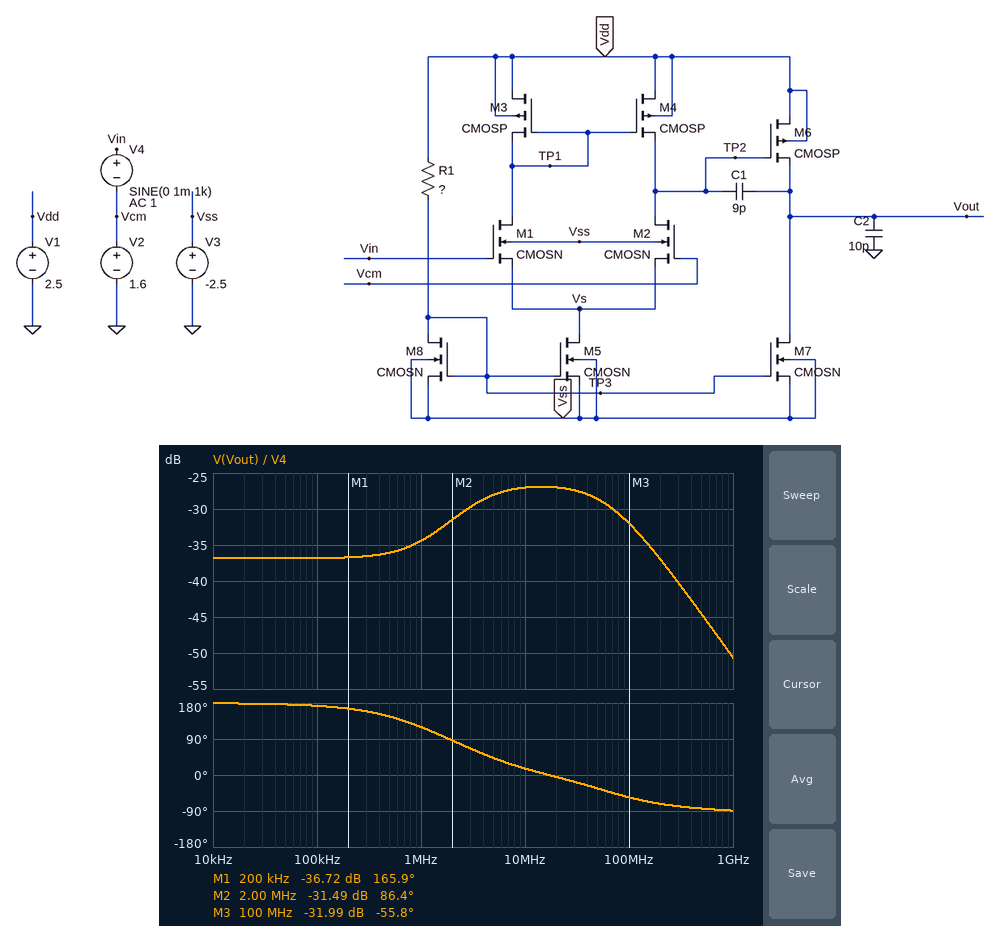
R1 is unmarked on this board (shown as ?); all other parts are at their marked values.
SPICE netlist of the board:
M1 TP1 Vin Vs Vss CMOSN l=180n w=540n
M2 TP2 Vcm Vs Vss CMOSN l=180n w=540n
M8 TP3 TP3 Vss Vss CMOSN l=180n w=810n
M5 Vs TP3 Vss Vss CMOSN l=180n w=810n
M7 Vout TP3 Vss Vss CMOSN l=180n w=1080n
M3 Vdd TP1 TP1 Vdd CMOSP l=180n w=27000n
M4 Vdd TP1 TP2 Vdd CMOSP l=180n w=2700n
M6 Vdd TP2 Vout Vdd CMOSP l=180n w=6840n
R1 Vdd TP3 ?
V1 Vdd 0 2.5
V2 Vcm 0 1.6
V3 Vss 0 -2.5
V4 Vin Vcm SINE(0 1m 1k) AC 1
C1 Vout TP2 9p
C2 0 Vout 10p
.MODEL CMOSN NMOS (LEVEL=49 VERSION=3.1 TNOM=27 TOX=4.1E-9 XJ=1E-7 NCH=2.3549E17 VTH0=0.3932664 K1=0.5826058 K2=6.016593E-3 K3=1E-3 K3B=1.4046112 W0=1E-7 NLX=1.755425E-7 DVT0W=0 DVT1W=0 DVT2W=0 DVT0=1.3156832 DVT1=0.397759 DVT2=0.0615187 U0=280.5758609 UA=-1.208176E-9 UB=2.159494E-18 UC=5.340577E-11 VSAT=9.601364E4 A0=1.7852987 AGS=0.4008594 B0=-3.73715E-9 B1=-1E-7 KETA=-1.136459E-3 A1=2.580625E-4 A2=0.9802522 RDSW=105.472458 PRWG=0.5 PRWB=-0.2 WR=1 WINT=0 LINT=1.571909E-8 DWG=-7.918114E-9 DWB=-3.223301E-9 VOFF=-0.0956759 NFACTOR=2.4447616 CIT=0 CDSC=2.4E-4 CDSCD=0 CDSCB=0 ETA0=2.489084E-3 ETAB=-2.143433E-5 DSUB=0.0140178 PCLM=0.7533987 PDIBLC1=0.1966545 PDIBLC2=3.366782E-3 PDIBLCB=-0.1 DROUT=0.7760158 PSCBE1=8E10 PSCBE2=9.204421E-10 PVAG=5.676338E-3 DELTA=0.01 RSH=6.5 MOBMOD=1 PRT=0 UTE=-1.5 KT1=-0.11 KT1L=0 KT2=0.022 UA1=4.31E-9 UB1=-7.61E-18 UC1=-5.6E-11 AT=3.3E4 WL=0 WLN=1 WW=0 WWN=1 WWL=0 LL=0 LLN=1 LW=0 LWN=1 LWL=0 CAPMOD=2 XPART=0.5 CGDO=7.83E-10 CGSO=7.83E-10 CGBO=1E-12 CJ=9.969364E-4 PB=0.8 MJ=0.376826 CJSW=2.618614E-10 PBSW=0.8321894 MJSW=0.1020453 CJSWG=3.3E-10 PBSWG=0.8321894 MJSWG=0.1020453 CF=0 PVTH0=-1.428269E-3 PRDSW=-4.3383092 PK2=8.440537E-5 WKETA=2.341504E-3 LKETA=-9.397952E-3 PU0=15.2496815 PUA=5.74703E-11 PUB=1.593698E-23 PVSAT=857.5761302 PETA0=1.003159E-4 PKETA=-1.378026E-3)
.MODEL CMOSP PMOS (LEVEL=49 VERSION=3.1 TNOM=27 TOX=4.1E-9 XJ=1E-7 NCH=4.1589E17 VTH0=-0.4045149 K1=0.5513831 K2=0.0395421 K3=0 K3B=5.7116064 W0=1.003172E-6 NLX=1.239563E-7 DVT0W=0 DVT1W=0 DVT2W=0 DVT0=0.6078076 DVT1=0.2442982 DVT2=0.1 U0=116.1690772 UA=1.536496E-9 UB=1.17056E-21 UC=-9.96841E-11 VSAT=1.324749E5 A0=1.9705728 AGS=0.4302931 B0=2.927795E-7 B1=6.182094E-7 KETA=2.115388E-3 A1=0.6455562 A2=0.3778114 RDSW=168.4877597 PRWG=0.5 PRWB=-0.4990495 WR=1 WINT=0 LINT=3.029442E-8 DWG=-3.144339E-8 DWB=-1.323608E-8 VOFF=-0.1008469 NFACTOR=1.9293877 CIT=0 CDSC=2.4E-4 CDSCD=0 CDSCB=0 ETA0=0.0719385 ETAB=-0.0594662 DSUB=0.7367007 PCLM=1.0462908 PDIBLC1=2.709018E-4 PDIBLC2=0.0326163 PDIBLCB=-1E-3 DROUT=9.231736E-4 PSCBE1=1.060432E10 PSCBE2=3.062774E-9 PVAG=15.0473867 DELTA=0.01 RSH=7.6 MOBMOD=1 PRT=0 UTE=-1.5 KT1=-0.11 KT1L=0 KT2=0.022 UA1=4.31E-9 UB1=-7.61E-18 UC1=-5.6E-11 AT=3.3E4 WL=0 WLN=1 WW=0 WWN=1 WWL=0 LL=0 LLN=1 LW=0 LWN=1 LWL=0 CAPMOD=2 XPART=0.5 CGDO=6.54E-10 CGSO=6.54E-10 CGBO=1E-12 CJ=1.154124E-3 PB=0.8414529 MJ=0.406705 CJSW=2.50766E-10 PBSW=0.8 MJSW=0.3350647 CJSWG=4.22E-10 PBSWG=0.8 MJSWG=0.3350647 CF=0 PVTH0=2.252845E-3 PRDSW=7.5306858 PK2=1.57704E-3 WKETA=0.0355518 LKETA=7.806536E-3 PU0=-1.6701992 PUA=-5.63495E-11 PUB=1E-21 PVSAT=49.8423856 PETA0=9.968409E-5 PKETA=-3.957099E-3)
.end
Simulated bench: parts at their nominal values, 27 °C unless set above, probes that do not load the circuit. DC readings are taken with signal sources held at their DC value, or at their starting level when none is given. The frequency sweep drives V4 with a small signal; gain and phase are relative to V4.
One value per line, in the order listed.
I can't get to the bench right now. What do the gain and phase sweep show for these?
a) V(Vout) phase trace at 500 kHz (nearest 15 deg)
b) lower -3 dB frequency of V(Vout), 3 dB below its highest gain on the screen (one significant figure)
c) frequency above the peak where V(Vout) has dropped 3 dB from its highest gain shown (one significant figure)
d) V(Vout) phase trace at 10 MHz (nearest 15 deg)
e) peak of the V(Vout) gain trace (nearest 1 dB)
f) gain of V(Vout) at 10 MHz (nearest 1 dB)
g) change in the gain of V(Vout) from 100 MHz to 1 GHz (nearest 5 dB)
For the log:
150 deg
3 MHz
70 MHz
15 deg
-27 dB
-27 dB
-20 dB
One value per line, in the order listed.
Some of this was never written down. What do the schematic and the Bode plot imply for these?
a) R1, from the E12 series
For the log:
33 kΩ
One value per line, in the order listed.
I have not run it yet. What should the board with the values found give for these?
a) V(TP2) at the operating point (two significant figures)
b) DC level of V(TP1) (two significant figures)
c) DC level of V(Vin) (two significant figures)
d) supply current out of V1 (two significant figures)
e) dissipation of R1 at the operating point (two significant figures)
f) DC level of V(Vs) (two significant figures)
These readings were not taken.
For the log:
140 mV
1.9 V
1.6 V
510 µA
500 µW
80 mV
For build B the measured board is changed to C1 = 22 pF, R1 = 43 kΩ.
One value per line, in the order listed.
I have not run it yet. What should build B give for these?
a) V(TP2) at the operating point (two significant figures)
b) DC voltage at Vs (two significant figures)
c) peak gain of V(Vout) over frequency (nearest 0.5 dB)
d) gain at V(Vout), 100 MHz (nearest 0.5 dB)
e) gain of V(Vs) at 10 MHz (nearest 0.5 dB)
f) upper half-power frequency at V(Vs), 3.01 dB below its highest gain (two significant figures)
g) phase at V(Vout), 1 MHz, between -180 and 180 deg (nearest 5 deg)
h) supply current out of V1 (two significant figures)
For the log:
200 mV
150 mV
-27.0 dB
-32.5 dB
-7.5 dB
1.9 MHz
75 deg
420 µA
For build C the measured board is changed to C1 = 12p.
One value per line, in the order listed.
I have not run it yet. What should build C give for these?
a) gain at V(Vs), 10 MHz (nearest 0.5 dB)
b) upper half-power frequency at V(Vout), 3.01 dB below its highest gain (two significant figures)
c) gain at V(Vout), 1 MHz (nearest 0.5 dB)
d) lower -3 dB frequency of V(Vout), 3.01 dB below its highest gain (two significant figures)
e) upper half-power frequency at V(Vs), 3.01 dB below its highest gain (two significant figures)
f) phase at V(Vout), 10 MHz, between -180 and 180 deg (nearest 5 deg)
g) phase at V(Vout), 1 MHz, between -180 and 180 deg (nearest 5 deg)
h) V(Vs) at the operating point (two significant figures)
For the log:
-7.5 dB
67 MHz
-33.5 dB
2.2 MHz
3.7 MHz
10 deg
105 deg
80 mV
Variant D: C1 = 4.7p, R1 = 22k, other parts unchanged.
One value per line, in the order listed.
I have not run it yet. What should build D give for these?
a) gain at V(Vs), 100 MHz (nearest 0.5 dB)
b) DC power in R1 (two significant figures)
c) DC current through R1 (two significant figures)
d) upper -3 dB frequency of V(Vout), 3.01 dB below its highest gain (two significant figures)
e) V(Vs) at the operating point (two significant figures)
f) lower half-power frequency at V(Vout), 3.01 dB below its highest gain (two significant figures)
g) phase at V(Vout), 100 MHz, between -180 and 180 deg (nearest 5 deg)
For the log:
-9.0 dB
700 µW
180 µA
77 MHz
-46 mV
5.4 MHz
-50 deg
